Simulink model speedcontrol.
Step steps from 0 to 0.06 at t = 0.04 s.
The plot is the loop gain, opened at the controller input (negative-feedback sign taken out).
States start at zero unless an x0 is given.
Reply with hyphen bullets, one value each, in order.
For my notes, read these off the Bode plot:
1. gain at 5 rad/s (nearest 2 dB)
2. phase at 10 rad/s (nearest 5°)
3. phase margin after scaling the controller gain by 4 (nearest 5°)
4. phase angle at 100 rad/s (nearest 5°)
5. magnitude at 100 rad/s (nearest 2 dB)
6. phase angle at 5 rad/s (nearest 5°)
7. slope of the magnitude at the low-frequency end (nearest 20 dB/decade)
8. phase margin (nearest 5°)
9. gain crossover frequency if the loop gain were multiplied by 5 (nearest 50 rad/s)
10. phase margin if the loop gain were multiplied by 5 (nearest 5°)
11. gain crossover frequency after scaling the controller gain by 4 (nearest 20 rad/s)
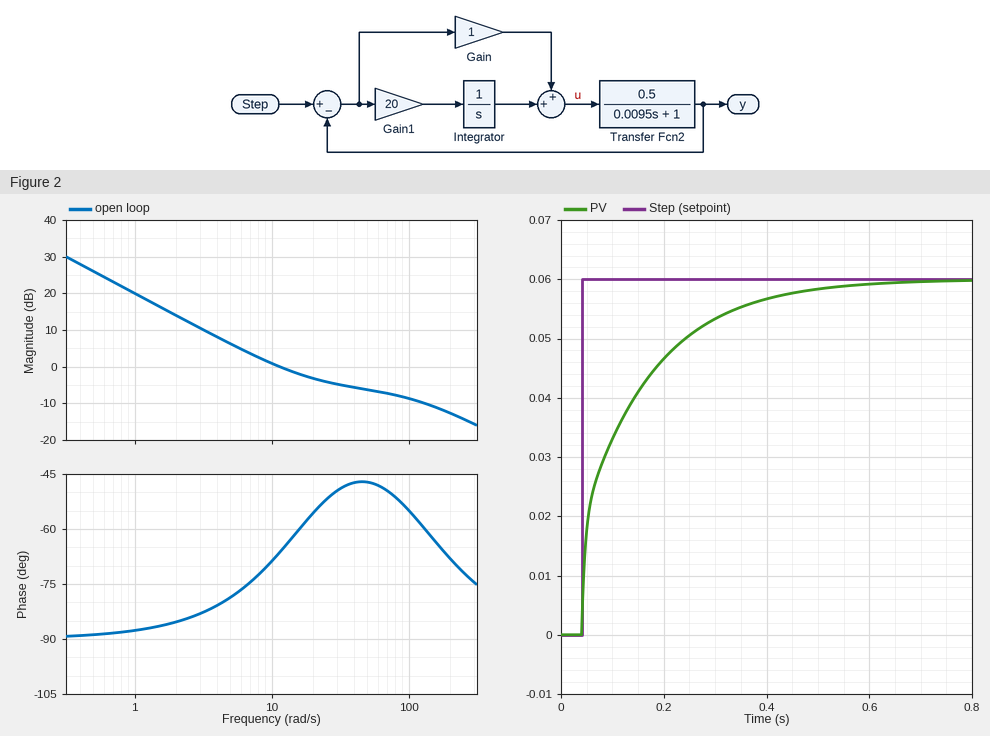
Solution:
- 6 dB
- -70°
- 115°
- -55°
- -8 dB
- -80°
- -20 dB/decade
- 115°
- 250 rad/s
- 110°
- 180 rad/s
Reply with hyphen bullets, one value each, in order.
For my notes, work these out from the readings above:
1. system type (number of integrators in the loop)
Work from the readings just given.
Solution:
- 1
